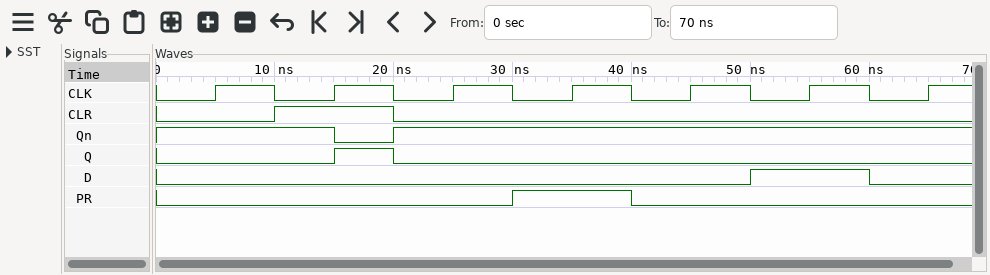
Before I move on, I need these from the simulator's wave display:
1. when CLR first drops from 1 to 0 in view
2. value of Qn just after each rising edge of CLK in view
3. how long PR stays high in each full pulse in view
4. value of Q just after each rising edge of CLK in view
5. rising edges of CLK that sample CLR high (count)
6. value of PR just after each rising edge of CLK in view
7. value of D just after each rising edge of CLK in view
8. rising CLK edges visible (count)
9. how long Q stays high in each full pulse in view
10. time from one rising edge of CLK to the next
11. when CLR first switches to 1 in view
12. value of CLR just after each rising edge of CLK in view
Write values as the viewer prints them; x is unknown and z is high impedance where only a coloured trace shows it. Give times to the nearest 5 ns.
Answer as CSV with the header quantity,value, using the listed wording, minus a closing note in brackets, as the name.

quantity,value
when CLR first drops from 1 to 0 in view,20 ns
value of Qn just after each rising edge of CLK in view,1 0 1 1 1 1 1
how long PR stays high in each full pulse in view,10 ns
value of Q just after each rising edge of CLK in view,0 1 0 0 0 0 0
rising edges of CLK that sample CLR high,1
value of PR just after each rising edge of CLK in view,0 0 0 1 0 0 0
value of D just after each rising edge of CLK in view,0 0 0 0 0 1 0
rising CLK edges visible,7
how long Q stays high in each full pulse in view,5 ns
time from one rising edge of CLK to the next,10 ns
when CLR first switches to 1 in view,10 ns
value of CLR just after each rising edge of CLK in view,0 1 0 0 0 0 0
